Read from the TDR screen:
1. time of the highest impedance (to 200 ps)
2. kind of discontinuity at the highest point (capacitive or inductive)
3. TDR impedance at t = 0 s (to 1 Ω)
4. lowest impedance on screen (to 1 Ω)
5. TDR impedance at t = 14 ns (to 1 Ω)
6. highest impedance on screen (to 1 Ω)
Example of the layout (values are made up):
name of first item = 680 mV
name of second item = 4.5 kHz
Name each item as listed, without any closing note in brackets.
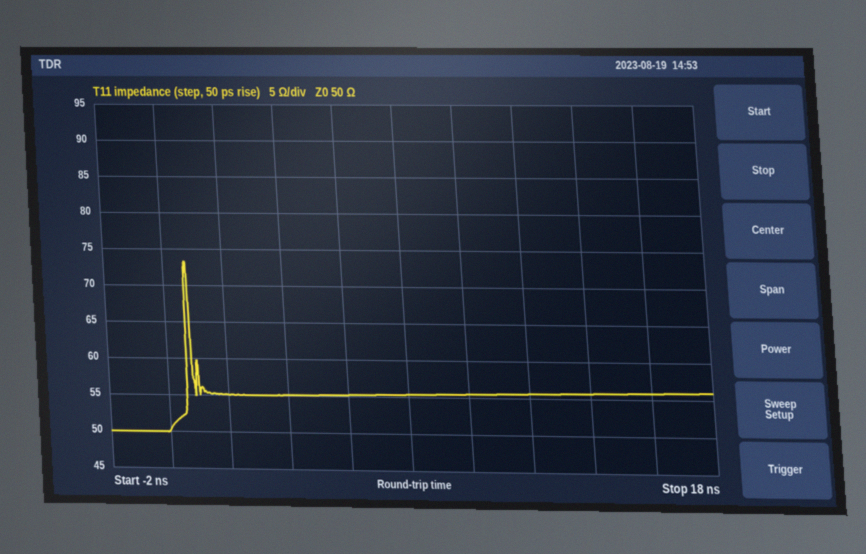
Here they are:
time of the highest impedance = 800 ps
kind of discontinuity at the highest point = inductive
TDR impedance at t = 0 s = 50 Ω
lowest impedance on screen = 50 Ω
TDR impedance at t = 14 ns = 56 Ω
highest impedance on screen = 73 Ω
